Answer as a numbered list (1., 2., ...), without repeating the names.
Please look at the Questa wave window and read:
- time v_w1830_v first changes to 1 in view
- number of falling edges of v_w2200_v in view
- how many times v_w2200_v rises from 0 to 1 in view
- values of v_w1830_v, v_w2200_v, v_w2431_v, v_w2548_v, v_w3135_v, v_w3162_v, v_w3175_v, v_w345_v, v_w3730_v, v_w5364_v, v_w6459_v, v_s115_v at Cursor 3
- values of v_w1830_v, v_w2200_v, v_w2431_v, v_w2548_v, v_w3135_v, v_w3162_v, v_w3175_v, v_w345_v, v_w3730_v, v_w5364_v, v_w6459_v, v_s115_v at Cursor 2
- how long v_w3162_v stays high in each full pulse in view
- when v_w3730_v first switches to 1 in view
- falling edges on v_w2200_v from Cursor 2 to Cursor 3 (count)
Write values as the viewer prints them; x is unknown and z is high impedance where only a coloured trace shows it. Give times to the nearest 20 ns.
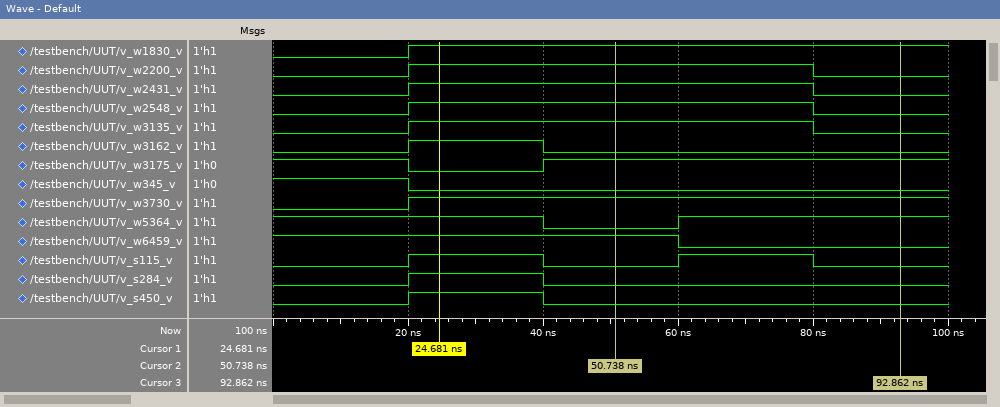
1. 20 ns
2. 1
3. 1
4. v_w1830_v=1, v_w2200_v=0, v_w2431_v=0, v_w2548_v=0, v_w3135_v=0, v_w3162_v=0, v_w3175_v=1, v_w345_v=0, v_w3730_v=1, v_w5364_v=1, v_w6459_v=0, v_s115_v=0
5. v_w1830_v=1, v_w2200_v=1, v_w2431_v=1, v_w2548_v=1, v_w3135_v=1, v_w3162_v=0, v_w3175_v=1, v_w345_v=0, v_w3730_v=1, v_w5364_v=0, v_w6459_v=1, v_s115_v=0
6. 20 ns
7. 20 ns
8. 1
